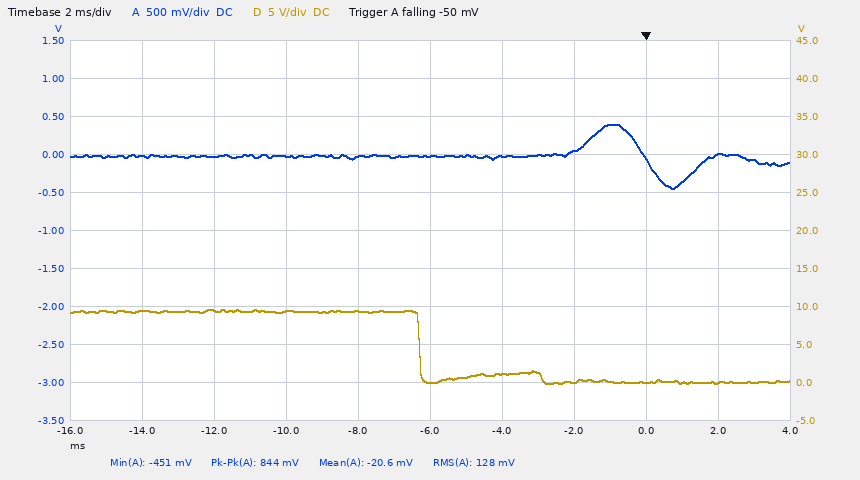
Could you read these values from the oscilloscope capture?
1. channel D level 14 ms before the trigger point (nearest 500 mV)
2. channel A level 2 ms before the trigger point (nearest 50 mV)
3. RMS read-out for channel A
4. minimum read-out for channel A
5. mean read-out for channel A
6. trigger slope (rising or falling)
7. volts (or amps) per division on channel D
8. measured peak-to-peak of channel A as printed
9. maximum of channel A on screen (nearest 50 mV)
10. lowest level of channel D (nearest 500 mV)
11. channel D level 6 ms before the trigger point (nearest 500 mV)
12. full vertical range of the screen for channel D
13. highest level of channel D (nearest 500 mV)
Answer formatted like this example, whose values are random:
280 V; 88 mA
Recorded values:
9.5 V; 50 mV; 128 mV; -451 mV; -20.6 mV; falling; 5 V; 844 mV; 400 mV; 0.0 V; 0.0 V; 50 V; 9.5 V
